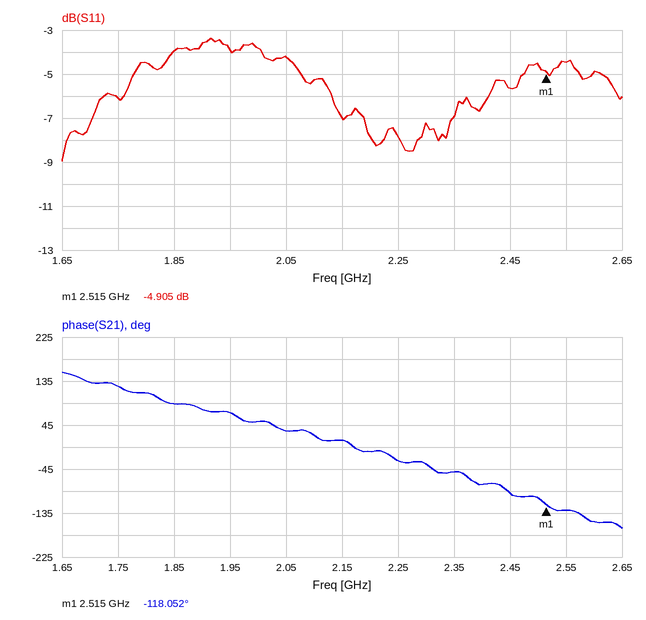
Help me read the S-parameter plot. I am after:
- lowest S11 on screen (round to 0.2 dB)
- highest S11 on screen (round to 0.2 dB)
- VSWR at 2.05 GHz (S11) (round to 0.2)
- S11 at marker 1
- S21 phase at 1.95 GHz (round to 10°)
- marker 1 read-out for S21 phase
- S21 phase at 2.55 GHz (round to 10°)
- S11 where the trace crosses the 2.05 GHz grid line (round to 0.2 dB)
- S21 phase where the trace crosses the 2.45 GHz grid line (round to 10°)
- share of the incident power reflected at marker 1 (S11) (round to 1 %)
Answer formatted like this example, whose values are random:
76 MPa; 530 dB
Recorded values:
-9.0 dB; -3.4 dB; 4.2; -4.905 dB; 70°; -118.052°; -130°; -4.2 dB; -90°; 32 %
